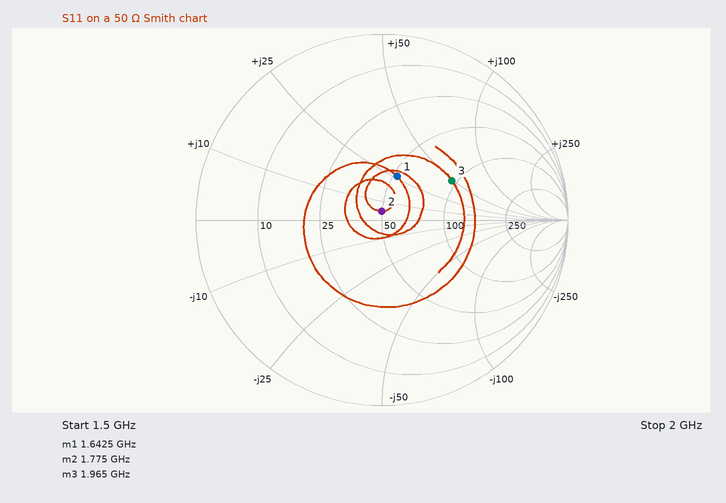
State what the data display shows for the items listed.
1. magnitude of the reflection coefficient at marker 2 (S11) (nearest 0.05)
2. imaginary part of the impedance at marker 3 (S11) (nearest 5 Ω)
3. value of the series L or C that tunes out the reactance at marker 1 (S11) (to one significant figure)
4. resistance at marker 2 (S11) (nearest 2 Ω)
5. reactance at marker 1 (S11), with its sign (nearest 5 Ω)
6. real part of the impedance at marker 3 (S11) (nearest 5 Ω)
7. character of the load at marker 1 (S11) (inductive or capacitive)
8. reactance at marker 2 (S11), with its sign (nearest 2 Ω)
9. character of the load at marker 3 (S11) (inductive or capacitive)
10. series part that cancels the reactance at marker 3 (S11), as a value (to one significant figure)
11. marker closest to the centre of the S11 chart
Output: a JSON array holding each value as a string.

["0.05", "+50 Ω", "4 pF", "50 Ω", "+25 Ω", "95 Ω", "inductive", "+4 Ω", "inductive", "2 pF", "marker 2"]
